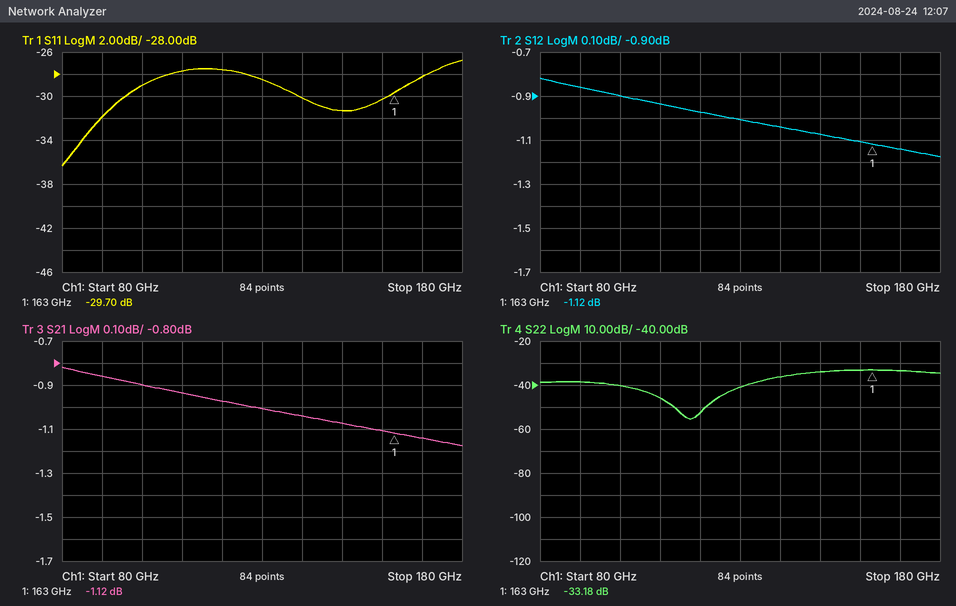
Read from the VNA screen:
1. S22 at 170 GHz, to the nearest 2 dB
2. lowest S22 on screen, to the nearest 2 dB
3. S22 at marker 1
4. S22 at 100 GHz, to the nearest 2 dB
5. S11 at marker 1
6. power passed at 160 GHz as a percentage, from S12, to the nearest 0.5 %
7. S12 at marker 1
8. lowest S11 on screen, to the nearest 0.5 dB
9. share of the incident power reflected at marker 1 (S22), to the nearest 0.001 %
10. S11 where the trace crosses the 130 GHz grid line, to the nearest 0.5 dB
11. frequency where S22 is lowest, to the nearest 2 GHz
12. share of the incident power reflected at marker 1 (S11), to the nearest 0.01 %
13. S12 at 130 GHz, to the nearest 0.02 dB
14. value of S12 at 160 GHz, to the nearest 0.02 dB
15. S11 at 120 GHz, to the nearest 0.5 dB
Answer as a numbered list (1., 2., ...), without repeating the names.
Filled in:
1. -34 dB
2. -56 dB
3. -33.18 dB
4. -40 dB
5. -29.70 dB
6. 77.5 %
7. -1.12 dB
8. -36.5 dB
9. 0.048 %
10. -28.5 dB
11. 118 GHz
12. 0.11 %
13. -1.00 dB
14. -1.10 dB
15. -27.5 dB
